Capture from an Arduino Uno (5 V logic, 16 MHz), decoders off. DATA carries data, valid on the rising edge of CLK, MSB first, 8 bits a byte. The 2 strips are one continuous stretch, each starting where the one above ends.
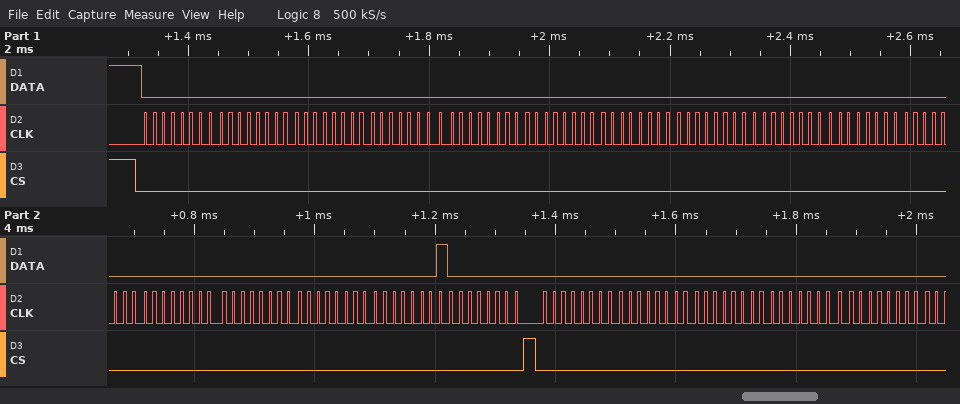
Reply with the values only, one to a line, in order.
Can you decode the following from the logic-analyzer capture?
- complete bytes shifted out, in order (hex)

00 00 00 00 00 00 00 00 00 00 00 00 00 00 01 00 00 00 00 00 00
